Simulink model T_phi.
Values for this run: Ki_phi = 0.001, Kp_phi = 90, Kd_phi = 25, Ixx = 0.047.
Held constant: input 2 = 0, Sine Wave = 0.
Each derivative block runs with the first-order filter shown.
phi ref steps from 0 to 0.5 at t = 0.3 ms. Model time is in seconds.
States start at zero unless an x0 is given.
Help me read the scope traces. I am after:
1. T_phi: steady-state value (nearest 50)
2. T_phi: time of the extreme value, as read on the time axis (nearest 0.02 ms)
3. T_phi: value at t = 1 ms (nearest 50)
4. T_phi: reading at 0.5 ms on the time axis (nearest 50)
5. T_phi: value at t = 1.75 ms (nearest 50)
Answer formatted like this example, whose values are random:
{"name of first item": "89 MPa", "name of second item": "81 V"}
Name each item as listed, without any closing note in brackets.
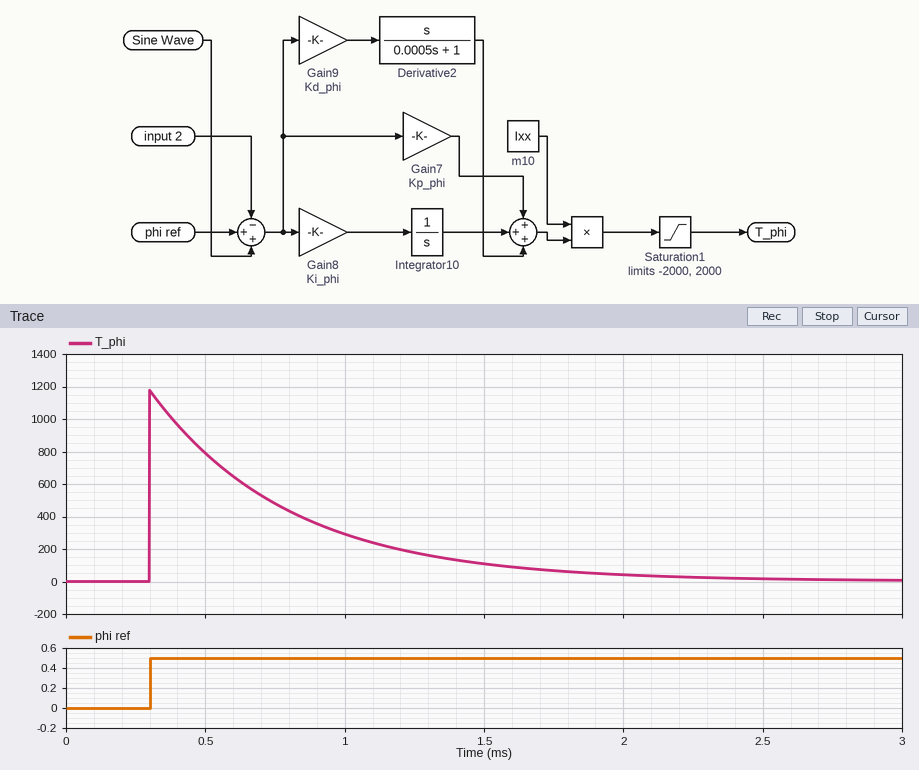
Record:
{"T_phi: steady-state value": "0", "T_phi: time of the extreme value, as read on the time axis": "0.30 ms", "T_phi: value at t = 1 ms": "300", "T_phi: reading at 0.5 ms on the time axis": "800", "T_phi: value at t = 1.75 ms": "50"}
